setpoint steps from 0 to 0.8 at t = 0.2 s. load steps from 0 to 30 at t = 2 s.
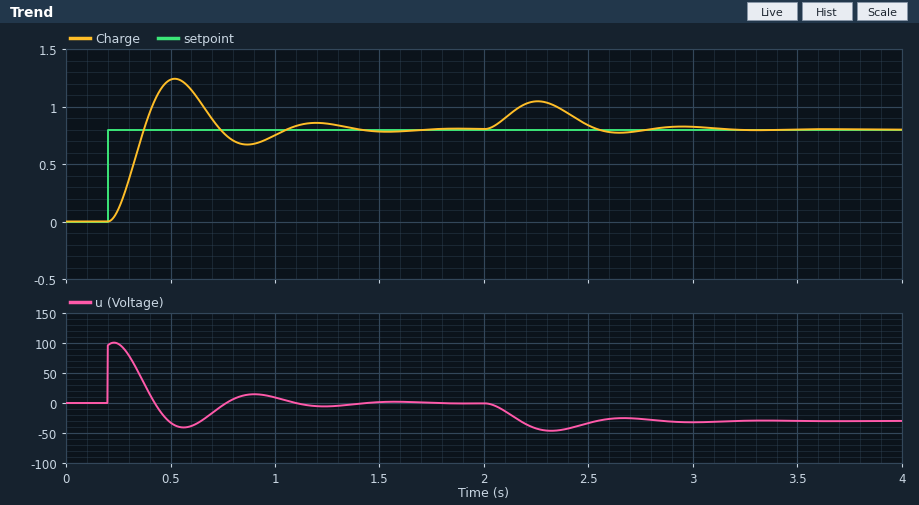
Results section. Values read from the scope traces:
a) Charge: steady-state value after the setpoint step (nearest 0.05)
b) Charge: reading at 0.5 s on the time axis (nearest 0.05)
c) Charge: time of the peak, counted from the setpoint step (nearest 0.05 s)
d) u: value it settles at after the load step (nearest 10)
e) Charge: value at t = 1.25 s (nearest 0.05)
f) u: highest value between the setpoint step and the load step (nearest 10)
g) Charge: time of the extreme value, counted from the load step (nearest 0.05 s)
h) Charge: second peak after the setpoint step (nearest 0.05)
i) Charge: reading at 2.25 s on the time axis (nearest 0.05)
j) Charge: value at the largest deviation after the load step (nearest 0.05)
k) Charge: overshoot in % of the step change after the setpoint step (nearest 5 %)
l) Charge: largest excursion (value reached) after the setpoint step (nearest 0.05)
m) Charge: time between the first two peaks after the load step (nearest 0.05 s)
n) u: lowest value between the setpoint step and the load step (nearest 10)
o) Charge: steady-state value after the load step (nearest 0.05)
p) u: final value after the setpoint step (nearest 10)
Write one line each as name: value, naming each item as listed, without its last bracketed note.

Charge: steady-state value after the setpoint step: 0.80
Charge: reading at 0.5 s on the time axis: 1.25
Charge: time of the peak, counted from the setpoint step: 0.30 s
u: value it settles at after the load step: -30
Charge: value at t = 1.25 s: 0.85
u: highest value between the setpoint step and the load step: 100
Charge: time of the extreme value, counted from the load step: 0.25 s
Charge: second peak after the setpoint step: 0.85
Charge: reading at 2.25 s on the time axis: 1.05
Charge: value at the largest deviation after the load step: 1.05
Charge: overshoot in % of the step change after the setpoint step: 55 %
Charge: largest excursion (value reached) after the setpoint step: 1.25
Charge: time between the first two peaks after the load step: 0.70 s
u: lowest value between the setpoint step and the load step: -40
Charge: steady-state value after the load step: 0.80
u: final value after the setpoint step: 0
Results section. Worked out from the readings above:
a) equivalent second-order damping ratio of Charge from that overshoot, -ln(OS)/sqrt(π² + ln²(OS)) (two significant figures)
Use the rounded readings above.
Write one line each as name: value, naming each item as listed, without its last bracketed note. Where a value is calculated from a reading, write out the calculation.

equivalent second-order damping ratio of Charge from that overshoot, -ln(OS)/sqrt(π² + ln²(OS)): ln(0.55) = -0.598; 0.598 / sqrt(9.870 + 0.357) = 0.19
